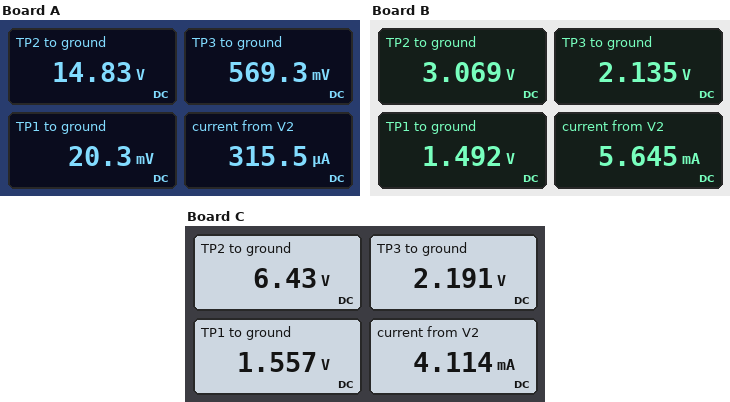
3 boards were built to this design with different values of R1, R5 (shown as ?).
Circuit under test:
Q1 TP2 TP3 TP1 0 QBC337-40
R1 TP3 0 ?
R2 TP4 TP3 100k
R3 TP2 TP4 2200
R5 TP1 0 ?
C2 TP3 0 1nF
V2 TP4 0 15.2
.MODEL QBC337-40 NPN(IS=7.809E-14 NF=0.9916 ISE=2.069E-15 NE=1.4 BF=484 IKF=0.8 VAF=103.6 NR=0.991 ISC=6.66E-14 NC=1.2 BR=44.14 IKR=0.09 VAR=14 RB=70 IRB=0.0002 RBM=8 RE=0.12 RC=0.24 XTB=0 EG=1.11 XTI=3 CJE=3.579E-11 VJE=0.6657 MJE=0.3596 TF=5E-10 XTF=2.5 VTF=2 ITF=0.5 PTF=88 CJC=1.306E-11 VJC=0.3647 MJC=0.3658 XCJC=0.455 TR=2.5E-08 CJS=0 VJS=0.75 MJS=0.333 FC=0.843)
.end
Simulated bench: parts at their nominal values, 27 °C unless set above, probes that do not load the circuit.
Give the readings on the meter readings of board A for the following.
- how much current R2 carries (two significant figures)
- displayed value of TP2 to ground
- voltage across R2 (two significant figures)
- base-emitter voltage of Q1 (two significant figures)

150 µA
14.83 V
15 V
550 mV
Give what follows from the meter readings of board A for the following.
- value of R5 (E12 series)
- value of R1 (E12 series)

120 Ω
3.9 kΩ
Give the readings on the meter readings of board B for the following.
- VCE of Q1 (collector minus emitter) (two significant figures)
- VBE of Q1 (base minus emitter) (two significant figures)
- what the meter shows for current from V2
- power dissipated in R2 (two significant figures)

1.6 V
640 mV
5.645 mA
1.7 mW
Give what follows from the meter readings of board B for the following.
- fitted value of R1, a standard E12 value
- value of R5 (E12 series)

18 kΩ
270 Ω
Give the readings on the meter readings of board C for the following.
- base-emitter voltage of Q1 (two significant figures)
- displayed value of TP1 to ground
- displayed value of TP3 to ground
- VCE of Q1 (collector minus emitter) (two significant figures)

630 mV
1.557 V
2.191 V
4.9 V
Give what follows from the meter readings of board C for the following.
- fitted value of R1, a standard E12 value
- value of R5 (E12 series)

18 kΩ
390 Ω
